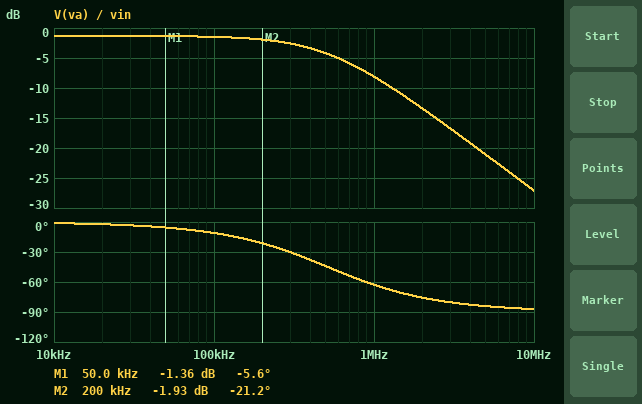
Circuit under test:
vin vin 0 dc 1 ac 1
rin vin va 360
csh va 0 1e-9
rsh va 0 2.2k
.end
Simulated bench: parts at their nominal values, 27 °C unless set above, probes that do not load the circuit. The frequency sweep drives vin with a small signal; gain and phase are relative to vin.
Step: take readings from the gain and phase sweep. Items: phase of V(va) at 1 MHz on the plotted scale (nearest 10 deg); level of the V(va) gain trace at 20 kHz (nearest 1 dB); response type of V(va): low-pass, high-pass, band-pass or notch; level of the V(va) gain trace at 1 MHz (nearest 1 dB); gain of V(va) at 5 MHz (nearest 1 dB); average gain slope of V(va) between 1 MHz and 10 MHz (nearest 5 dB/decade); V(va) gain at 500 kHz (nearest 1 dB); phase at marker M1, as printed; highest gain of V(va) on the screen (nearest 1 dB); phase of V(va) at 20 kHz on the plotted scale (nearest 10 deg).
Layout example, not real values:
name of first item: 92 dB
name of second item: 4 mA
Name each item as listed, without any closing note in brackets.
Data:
phase of V(va) at 1 MHz on the plotted scale: -60 deg
level of the V(va) gain trace at 20 kHz: -1 dB
response type of V(va): low-pass, high-pass, band-pass or notch: low-pass
level of the V(va) gain trace at 1 MHz: -8 dB
gain of V(va) at 5 MHz: -21 dB
average gain slope of V(va) between 1 MHz and 10 MHz: -20 dB/decade
V(va) gain at 500 kHz: -4 dB
phase at marker M1, as printed: -5.6 deg
highest gain of V(va) on the screen: -1 dB
phase of V(va) at 20 kHz on the plotted scale: 0 deg
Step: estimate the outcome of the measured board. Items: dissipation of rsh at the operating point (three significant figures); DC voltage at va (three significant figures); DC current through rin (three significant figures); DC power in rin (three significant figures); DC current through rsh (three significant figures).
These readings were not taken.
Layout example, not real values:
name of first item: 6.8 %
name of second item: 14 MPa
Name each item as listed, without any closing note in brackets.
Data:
dissipation of rsh at the operating point: 336 µW
DC voltage at va: 859 mV
DC current through rin: 391 µA
DC power in rin: 54.9 µW
DC current through rsh: 391 µA
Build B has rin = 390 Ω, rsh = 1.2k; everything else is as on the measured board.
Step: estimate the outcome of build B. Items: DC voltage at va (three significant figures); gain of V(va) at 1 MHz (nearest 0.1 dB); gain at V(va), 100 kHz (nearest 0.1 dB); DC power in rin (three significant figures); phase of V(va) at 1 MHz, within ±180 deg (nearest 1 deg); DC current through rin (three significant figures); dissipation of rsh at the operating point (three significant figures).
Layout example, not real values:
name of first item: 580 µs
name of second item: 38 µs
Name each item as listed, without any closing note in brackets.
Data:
DC voltage at va: 755 mV
gain of V(va) at 1 MHz: -8.9 dB
gain at V(va), 100 kHz: -2.6 dB
DC power in rin: 154 µW
phase of V(va) at 1 MHz, within ±180 deg: -62 deg
DC current through rin: 629 µA
dissipation of rsh at the operating point: 475 µW
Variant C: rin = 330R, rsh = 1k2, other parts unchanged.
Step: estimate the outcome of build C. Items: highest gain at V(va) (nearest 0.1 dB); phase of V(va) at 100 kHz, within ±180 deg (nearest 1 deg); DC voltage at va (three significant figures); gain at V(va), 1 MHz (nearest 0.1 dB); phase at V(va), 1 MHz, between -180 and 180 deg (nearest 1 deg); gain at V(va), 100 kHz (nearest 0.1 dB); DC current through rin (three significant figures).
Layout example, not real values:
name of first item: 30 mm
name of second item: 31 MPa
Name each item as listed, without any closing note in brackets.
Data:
highest gain at V(va): -2.1 dB
phase of V(va) at 100 kHz, within ±180 deg: -9 deg
DC voltage at va: 784 mV
gain at V(va), 1 MHz: -7.7 dB
phase at V(va), 1 MHz, between -180 and 180 deg: -58 deg
gain at V(va), 100 kHz: -2.2 dB
DC current through rin: 654 µA
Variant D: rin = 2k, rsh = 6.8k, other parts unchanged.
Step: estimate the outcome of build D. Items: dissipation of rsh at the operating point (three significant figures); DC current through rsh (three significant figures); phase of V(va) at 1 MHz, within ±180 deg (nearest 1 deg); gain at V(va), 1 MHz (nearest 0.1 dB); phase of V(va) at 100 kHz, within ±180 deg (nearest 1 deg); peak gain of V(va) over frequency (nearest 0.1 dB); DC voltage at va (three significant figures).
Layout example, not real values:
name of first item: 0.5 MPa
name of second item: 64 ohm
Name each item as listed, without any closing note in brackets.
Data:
dissipation of rsh at the operating point: 87.8 µW
DC current through rsh: 114 µA
phase of V(va) at 1 MHz, within ±180 deg: -84 deg
gain at V(va), 1 MHz: -22.0 dB
phase of V(va) at 100 kHz, within ±180 deg: -44 deg
peak gain of V(va) over frequency: -2.2 dB
DC voltage at va: 773 mV
